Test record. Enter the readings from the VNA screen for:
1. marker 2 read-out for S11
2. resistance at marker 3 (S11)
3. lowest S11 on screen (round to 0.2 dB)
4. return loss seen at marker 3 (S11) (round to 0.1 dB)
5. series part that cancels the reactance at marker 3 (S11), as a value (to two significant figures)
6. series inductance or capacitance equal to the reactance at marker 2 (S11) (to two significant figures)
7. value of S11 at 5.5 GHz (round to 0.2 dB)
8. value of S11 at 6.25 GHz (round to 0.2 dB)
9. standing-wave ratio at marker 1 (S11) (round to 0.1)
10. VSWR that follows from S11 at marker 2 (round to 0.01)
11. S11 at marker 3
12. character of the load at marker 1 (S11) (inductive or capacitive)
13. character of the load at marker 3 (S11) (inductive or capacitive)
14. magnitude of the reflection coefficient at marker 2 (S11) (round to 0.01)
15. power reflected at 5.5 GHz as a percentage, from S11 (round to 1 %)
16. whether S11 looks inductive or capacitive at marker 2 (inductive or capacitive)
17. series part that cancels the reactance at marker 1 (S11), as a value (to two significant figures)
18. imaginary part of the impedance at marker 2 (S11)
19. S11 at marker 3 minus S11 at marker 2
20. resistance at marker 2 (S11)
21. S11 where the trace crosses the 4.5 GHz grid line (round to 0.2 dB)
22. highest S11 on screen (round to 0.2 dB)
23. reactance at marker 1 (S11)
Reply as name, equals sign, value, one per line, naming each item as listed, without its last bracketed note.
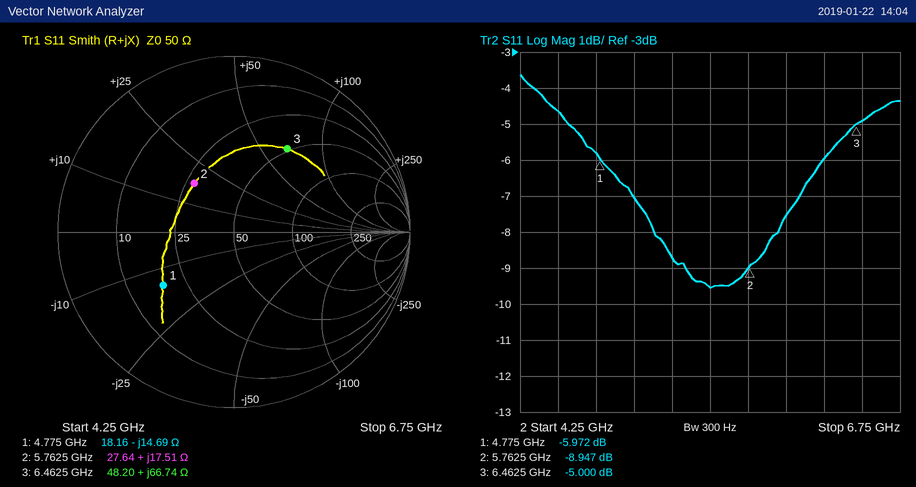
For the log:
marker 2 read-out for S11 = -8.947 dB
resistance at marker 3 = 48.20 Ω
lowest S11 on screen = -9.6 dB
return loss seen at marker 3 (S11) = 5.0 dB
series part that cancels the reactance at marker 3 (S11), as a value = 370 fF
series inductance or capacitance equal to the reactance at marker 2 (S11) = 480 pH
value of S11 at 5.5 GHz = -9.6 dB
value of S11 at 6.25 GHz = -6.0 dB
standing-wave ratio at marker 1 (S11) = 3.0
VSWR that follows from S11 at marker 2 = 2.11
S11 at marker 3 = -5.000 dB
character of the load at marker 1 (S11) = capacitive
character of the load at marker 3 (S11) = inductive
magnitude of the reflection coefficient at marker 2 (S11) = 0.36
power reflected at 5.5 GHz as a percentage, from S11 = 11 %
whether S11 looks inductive or capacitive at marker 2 = inductive
series part that cancels the reactance at marker 1 (S11), as a value = 490 pH
imaginary part of the impedance at marker 2 = +17.51 Ω
S11 at marker 3 minus S11 at marker 2 = 3.947 dB
resistance at marker 2 = 27.64 Ω
S11 where the trace crosses the 4.5 GHz grid line = -4.6 dB
highest S11 on screen = -3.6 dB
reactance at marker 1 = -14.69 Ω
